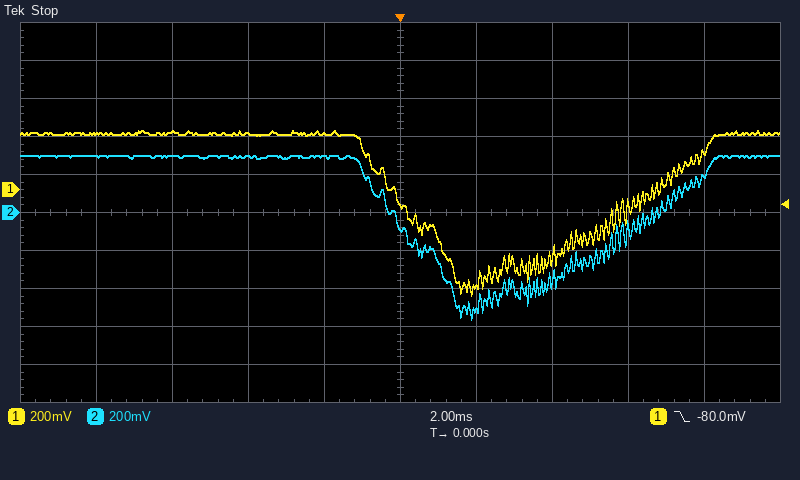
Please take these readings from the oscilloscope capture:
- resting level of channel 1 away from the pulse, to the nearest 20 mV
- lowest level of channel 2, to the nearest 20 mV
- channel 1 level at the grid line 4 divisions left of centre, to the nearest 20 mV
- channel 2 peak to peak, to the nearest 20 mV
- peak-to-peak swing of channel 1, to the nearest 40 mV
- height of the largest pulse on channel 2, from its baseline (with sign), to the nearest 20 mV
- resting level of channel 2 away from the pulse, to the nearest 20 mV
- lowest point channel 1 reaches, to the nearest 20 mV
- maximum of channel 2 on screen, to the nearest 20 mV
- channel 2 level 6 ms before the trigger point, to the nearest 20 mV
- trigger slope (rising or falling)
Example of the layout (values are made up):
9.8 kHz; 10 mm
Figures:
300 mV; -560 mV; 300 mV; 860 mV; 880 mV; -860 mV; 300 mV; -560 mV; 300 mV; 300 mV; falling
